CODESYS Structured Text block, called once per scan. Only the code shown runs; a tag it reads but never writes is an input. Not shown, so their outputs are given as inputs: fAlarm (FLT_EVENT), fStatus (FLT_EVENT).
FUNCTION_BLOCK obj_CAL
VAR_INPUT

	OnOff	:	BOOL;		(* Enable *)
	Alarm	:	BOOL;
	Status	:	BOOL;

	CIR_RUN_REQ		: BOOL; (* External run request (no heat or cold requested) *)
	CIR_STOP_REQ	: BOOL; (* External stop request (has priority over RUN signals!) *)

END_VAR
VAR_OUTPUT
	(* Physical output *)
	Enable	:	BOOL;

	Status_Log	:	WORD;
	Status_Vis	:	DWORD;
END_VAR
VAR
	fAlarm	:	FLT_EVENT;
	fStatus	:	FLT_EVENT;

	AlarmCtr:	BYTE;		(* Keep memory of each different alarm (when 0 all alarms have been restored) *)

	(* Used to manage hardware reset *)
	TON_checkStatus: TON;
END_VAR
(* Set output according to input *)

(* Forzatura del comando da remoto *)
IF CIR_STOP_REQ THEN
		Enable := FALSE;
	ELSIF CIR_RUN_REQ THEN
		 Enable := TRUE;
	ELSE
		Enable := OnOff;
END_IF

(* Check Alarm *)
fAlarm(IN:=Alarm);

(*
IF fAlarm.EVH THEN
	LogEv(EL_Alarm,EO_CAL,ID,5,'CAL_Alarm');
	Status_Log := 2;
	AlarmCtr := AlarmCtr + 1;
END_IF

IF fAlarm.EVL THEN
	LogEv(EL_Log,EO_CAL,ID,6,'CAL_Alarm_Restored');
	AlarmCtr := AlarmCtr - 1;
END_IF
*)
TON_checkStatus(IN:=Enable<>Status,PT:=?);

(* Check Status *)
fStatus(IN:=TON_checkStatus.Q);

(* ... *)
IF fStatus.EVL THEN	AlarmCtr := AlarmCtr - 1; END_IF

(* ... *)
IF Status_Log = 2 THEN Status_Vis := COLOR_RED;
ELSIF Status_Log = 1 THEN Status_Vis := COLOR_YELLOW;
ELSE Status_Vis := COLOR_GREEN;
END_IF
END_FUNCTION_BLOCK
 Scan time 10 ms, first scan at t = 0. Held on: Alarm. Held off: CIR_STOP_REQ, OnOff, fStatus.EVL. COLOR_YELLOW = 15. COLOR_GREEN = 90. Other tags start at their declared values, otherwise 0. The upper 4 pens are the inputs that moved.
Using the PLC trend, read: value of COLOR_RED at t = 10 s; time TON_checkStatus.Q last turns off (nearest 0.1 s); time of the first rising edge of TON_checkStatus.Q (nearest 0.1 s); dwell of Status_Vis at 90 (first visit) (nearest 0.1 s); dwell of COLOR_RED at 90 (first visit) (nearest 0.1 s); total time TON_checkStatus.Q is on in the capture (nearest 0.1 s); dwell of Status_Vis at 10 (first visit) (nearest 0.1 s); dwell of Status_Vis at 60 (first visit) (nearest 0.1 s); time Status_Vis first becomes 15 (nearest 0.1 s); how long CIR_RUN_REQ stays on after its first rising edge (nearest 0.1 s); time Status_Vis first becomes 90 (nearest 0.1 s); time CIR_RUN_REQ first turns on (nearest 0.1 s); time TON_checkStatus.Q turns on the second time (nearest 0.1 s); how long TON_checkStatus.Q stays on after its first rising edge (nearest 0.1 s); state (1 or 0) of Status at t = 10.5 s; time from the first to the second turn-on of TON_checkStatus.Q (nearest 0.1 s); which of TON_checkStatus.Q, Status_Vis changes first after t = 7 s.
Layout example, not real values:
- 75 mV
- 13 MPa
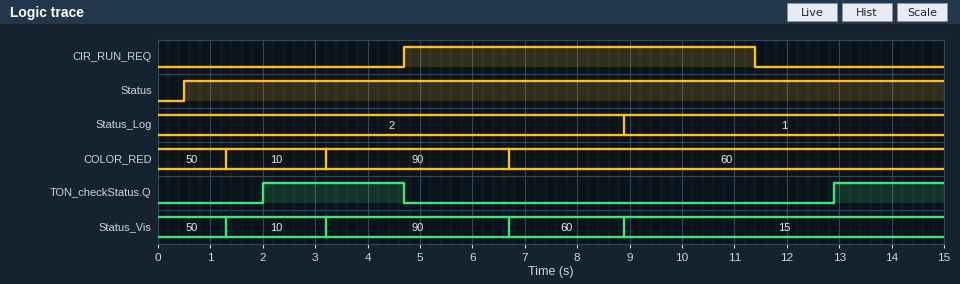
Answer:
- 60
- 4.7 s
- 2.0 s
- 3.5 s
- 3.5 s
- 4.8 s
- 1.9 s
- 2.2 s
- 8.9 s
- 6.7 s
- 3.2 s
- 4.7 s
- 12.9 s
- 2.7 s
- 1
- 10.9 s
- Status_Vis
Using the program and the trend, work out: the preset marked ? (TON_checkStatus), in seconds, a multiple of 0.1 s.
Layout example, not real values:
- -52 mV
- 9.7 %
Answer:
- 1.5 s
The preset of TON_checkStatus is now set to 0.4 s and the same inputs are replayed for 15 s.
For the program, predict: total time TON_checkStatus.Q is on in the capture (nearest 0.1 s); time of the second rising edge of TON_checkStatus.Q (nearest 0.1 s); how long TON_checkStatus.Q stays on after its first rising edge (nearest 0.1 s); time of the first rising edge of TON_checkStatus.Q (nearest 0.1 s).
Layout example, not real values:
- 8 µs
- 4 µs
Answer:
- 7.0 s
- 11.8 s
- 3.8 s
- 0.9 s
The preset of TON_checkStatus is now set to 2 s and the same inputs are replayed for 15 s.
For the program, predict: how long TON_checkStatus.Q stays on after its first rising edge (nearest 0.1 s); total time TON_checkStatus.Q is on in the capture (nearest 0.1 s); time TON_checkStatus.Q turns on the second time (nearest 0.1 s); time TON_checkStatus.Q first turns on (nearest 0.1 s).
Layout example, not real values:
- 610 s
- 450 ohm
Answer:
- 2.2 s
- 3.8 s
- 13.4 s
- 2.5 s
